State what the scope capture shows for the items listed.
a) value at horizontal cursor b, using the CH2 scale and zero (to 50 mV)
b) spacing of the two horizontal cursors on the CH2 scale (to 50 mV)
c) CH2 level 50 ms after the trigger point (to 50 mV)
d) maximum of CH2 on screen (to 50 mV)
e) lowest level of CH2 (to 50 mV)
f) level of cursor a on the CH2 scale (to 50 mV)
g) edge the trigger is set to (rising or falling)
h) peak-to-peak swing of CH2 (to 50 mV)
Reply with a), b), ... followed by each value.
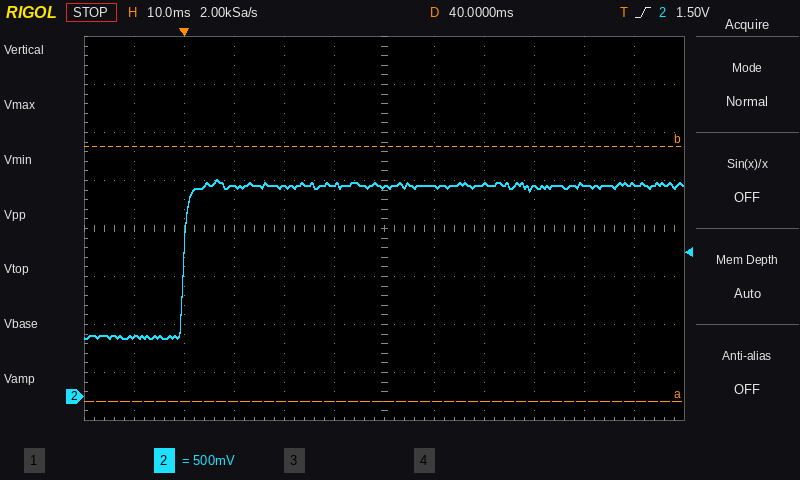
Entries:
a) 2.60 V
b) 2.65 V
c) 2.20 V
d) 2.25 V
e) 600 mV
f) -50 mV
g) rising
h) 1.65 V
